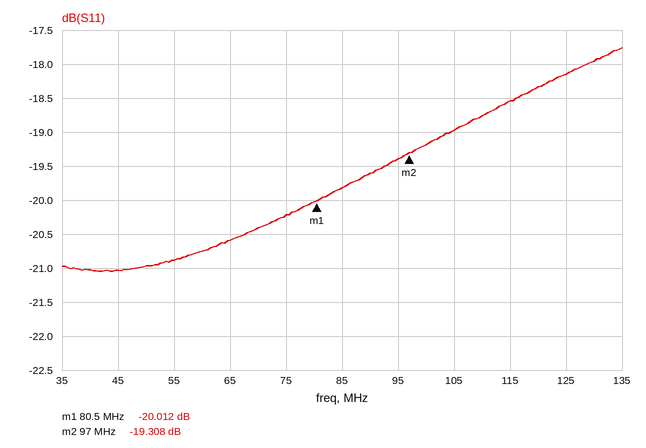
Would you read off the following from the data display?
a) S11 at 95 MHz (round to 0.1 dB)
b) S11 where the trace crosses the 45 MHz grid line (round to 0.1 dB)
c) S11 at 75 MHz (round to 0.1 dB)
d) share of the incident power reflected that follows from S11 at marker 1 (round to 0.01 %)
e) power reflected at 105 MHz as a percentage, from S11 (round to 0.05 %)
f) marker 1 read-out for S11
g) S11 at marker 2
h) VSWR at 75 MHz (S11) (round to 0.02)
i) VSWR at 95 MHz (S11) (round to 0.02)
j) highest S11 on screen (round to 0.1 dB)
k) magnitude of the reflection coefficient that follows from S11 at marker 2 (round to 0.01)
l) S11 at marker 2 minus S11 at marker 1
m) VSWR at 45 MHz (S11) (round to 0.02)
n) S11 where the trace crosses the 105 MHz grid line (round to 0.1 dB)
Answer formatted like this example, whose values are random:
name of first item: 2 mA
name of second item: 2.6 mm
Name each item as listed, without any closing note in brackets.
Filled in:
S11 at 95 MHz: -19.4 dB
S11 where the trace crosses the 45 MHz grid line: -21.0 dB
S11 at 75 MHz: -20.2 dB
share of the incident power reflected that follows from S11 at marker 1: 1.00 %
power reflected at 105 MHz as a percentage, from S11: 1.25 %
marker 1 read-out for S11: -20.012 dB
S11 at marker 2: -19.308 dB
VSWR at 75 MHz (S11): 1.22
VSWR at 95 MHz (S11): 1.24
highest S11 on screen: -17.8 dB
magnitude of the reflection coefficient that follows from S11 at marker 2: 0.11
S11 at marker 2 minus S11 at marker 1: 0.704 dB
VSWR at 45 MHz (S11): 1.20
S11 where the trace crosses the 105 MHz grid line: -19.0 dB
